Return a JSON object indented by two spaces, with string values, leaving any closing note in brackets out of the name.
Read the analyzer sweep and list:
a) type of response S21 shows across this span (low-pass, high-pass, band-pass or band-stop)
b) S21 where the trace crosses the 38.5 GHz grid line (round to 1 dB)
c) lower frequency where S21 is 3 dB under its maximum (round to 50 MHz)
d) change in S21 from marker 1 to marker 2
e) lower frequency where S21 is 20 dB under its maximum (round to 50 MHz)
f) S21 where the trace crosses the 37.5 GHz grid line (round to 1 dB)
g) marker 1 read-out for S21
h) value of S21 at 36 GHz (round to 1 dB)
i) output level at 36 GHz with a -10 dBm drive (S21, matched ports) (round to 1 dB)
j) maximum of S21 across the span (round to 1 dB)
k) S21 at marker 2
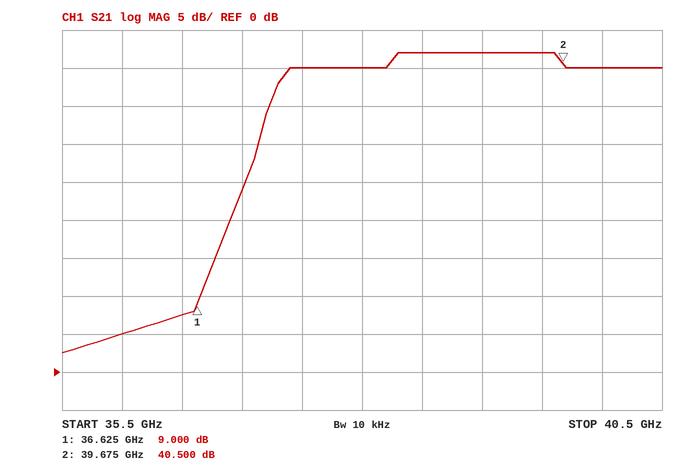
{
  "type of response S21 shows across this span": "high-pass",
  "S21 where the trace crosses the 38.5 GHz grid line": "42 dB",
  "lower frequency where S21 is 3 dB under its maximum": "37.35 GHz",
  "change in S21 from marker 1 to marker 2": "31.500 dB",
  "lower frequency where S21 is 20 dB under its maximum": "36.95 GHz",
  "S21 where the trace crosses the 37.5 GHz grid line": "40 dB",
  "marker 1 read-out for S21": "9.000 dB",
  "value of S21 at 36 GHz": "5 dB",
  "output level at 36 GHz with a -10 dBm drive (S21, matched ports)": "-5 dBm",
  "maximum of S21 across the span": "42 dB",
  "S21 at marker 2": "40.500 dB"
}
